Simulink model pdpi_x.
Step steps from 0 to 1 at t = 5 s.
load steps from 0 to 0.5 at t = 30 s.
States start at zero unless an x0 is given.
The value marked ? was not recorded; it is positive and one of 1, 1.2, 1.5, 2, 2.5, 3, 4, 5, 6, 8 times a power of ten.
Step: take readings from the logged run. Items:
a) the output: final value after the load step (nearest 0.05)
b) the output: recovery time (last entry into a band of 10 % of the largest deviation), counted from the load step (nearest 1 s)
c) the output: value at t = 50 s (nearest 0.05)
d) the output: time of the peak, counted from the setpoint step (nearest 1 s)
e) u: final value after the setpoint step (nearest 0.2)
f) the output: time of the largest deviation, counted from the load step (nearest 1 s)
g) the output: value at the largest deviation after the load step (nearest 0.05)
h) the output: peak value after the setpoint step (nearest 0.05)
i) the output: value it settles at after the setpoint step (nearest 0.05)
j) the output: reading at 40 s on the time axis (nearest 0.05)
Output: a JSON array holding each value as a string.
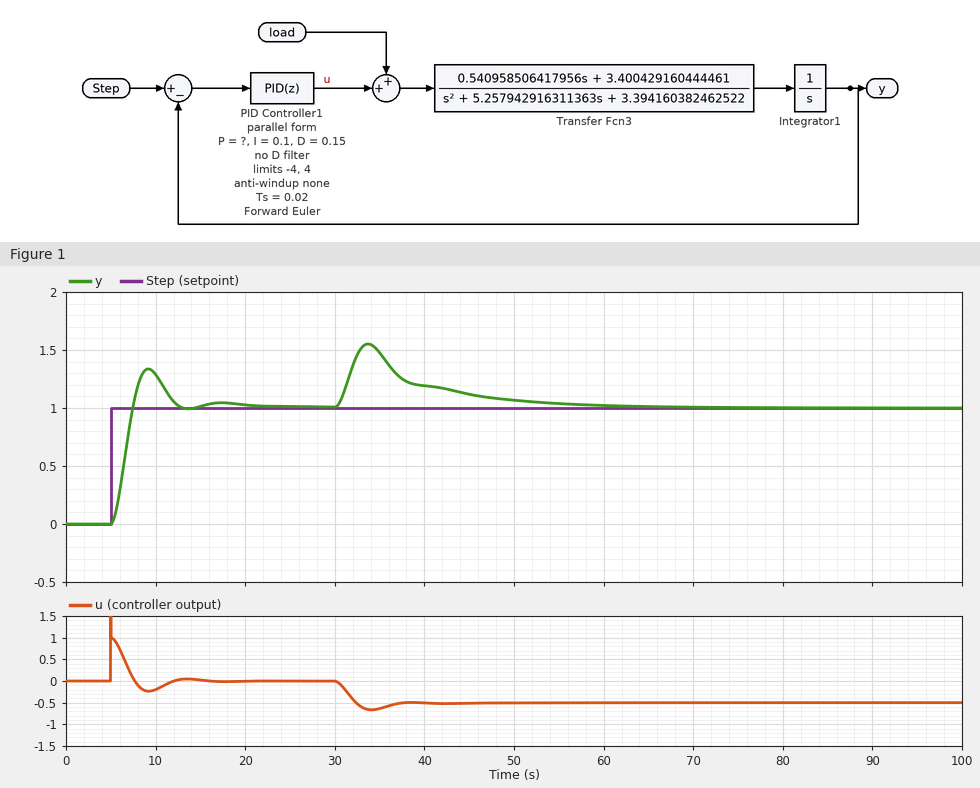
["1.00", "22 s", "1.05", "4 s", "0.0", "4 s", "1.55", "1.35", "1.00", "1.20"]
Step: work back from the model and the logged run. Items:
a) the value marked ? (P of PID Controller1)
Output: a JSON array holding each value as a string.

["1"]
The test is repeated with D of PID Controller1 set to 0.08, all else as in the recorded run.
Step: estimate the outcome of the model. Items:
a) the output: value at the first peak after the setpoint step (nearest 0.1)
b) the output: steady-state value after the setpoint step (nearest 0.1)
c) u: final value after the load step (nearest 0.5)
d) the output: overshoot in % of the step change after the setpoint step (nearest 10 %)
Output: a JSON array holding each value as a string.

["1.4", "1.0", "-0.5", "40 %"]
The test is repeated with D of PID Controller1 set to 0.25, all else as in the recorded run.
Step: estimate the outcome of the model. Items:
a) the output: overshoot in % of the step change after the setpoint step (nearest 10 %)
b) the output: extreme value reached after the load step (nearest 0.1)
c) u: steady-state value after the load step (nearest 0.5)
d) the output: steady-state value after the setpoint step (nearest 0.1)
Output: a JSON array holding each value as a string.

["30 %", "1.5", "-0.5", "1.0"]
